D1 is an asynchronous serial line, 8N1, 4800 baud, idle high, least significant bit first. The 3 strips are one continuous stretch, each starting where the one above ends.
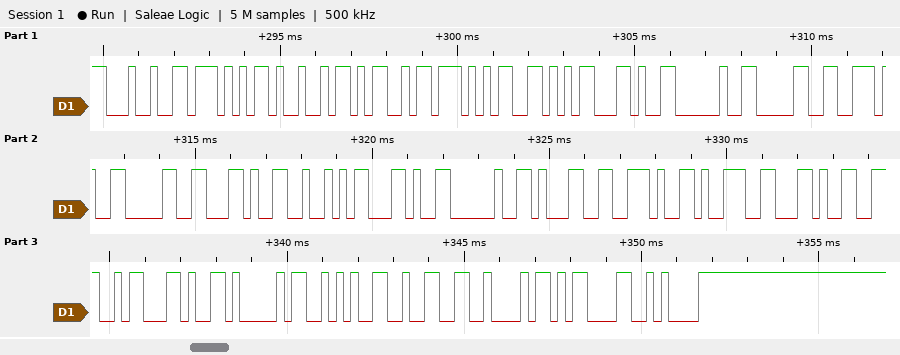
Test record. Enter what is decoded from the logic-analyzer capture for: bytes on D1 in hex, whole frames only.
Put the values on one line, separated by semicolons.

24 57 49 4D 57 56 2C 20 30 2E 30 2C 52 2C 20 31 2E 39 2C 4E 2C 41 2A 32 42 0D 0A
